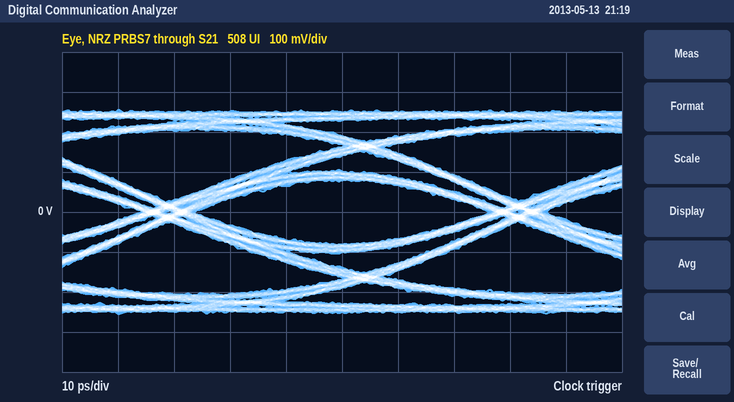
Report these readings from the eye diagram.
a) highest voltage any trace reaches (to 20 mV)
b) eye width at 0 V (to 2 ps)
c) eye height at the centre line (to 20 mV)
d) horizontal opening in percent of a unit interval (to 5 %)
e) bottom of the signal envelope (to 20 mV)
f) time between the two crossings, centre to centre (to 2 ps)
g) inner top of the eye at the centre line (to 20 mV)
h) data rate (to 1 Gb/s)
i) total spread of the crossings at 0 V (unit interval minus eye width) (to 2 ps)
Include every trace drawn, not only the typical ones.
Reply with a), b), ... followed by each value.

a) 260 mV
b) 52 ps
c) 160 mV
d) 85 %
e) -260 mV
f) 62 ps
g) 80 mV
h) 16 Gb/s
i) 10 ps
